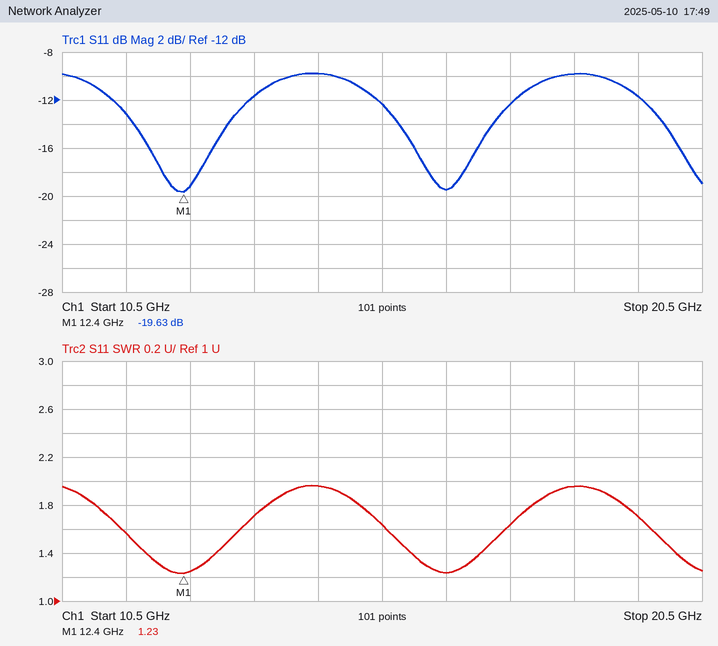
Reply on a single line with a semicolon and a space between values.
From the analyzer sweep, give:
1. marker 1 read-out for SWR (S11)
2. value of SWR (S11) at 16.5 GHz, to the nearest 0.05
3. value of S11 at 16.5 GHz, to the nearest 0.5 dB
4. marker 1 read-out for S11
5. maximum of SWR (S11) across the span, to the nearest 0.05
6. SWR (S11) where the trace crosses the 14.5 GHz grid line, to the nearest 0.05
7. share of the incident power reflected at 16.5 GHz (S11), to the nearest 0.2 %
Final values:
1.23; 1.25; -19.5 dB; -19.63 dB; 1.95; 1.95; 1.2 %
